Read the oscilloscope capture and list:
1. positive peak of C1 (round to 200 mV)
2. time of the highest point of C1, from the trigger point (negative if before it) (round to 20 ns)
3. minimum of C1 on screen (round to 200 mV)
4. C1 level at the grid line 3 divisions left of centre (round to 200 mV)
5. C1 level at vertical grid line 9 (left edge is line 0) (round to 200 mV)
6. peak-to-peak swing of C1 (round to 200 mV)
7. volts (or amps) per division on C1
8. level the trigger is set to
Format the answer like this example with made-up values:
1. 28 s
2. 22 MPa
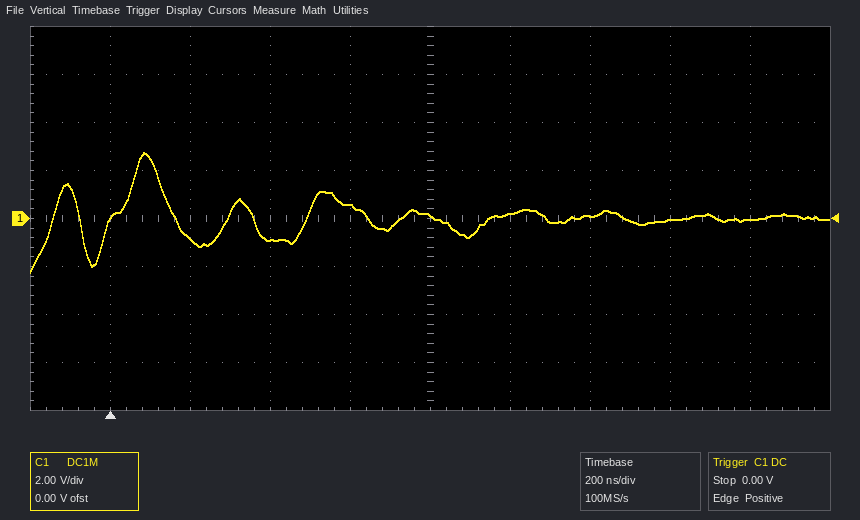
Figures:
1. 2.8 V
2. +80 ns
3. -2.2 V
4. -800 mV
5. 0.0 V
6. 5.0 V
7. 2 V
8. 0.00 V
